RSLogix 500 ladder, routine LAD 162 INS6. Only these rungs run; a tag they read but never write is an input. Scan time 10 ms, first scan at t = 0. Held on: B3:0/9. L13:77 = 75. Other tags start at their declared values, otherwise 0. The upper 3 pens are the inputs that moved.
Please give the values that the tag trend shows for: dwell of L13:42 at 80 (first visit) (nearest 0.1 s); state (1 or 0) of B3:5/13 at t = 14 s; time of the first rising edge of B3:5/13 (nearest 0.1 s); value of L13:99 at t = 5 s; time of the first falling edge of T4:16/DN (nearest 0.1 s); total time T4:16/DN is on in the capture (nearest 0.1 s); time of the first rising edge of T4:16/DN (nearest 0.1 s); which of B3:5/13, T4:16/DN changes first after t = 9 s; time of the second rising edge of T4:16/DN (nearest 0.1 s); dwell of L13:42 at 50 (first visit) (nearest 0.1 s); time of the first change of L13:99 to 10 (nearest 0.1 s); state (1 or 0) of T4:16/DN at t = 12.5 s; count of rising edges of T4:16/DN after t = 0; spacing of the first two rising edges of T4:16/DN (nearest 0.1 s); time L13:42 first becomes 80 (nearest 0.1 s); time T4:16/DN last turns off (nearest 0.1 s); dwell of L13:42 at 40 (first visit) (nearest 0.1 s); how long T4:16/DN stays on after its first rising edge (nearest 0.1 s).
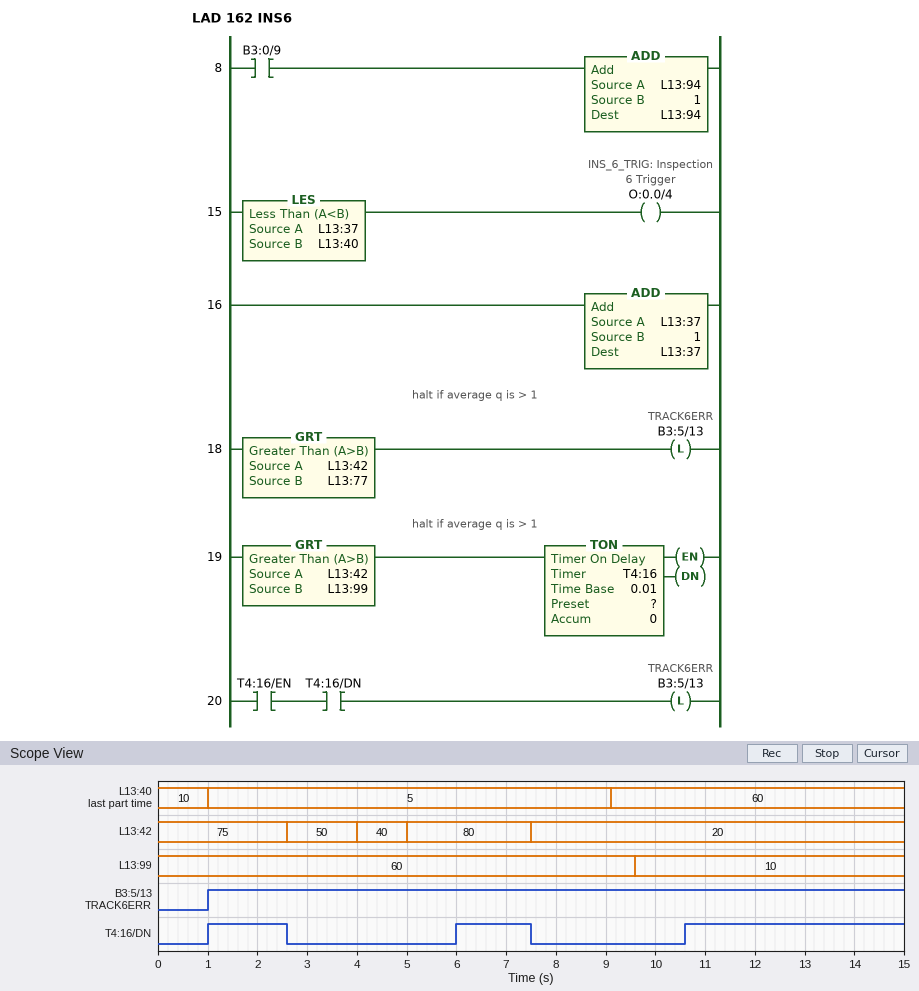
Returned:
2.5 s
1
1.0 s
60
2.6 s
7.5 s
1.0 s
T4:16/DN
6.0 s
1.4 s
9.6 s
1
3
5.0 s
5.0 s
7.5 s
1.0 s
1.6 s
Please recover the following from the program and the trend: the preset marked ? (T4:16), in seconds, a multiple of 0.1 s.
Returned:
1.0 s
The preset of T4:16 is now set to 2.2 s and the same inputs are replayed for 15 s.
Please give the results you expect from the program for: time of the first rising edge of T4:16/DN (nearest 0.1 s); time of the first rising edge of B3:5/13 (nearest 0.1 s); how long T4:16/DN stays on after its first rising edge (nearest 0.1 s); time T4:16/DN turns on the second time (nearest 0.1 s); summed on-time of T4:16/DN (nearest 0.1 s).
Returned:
2.2 s
2.2 s
0.4 s
7.2 s
3.9 s
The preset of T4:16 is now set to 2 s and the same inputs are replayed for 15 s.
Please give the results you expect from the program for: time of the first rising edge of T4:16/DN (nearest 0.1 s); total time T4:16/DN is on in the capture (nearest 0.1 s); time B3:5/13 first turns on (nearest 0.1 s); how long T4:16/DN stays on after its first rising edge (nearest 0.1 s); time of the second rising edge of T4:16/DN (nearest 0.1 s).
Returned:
2.0 s
4.5 s
2.0 s
0.6 s
7.0 s
